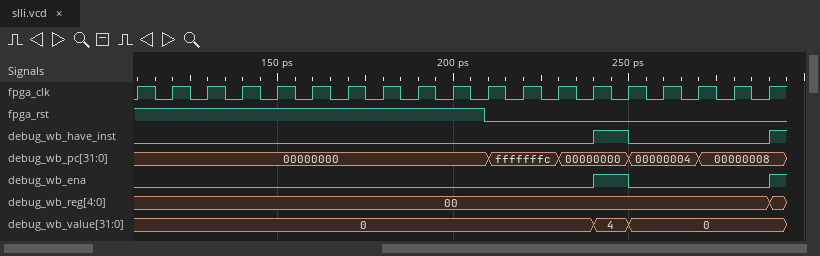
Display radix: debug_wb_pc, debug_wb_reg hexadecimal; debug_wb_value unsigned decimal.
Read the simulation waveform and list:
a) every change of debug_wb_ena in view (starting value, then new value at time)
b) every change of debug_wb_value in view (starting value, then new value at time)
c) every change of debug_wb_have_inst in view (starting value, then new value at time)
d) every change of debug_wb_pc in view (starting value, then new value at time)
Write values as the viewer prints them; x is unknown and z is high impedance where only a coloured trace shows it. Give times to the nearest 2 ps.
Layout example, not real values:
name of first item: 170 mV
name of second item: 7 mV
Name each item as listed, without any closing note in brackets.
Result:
every change of debug_wb_ena in view: 0, 1 at 240 ps, 0 at 250 ps, 1 at 290 ps
every change of debug_wb_value in view: 0, 4 at 240 ps, 0 at 250 ps
every change of debug_wb_have_inst in view: 0, 1 at 240 ps, 0 at 250 ps, 1 at 290 ps
every change of debug_wb_pc in view: 00000000, fffffffc at 210 ps, 00000000 at 230 ps, 00000004 at 250 ps, 00000008 at 270 ps
